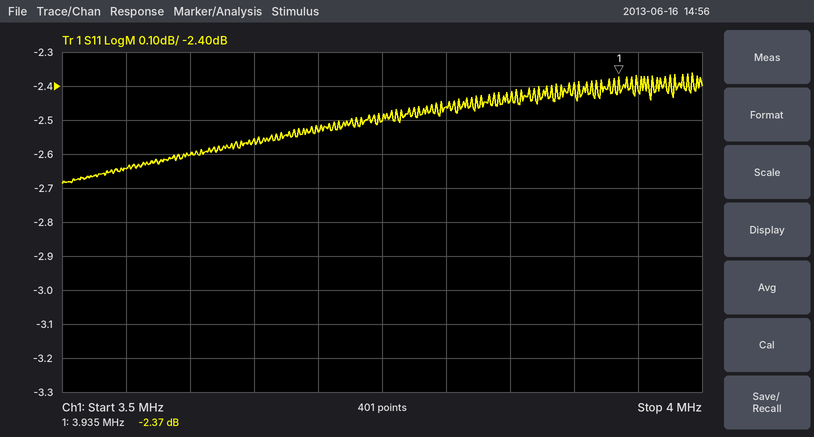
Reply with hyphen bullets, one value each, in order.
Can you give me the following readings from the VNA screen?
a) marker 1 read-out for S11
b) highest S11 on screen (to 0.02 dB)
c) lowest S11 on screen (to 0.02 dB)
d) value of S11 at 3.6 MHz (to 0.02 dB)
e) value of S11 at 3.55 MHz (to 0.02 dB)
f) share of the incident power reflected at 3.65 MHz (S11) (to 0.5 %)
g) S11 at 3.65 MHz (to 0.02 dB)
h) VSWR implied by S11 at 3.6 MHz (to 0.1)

- -2.37 dB
- -2.36 dB
- -2.68 dB
- -2.60 dB
- -2.64 dB
- 55.5 %
- -2.56 dB
- 6.7
